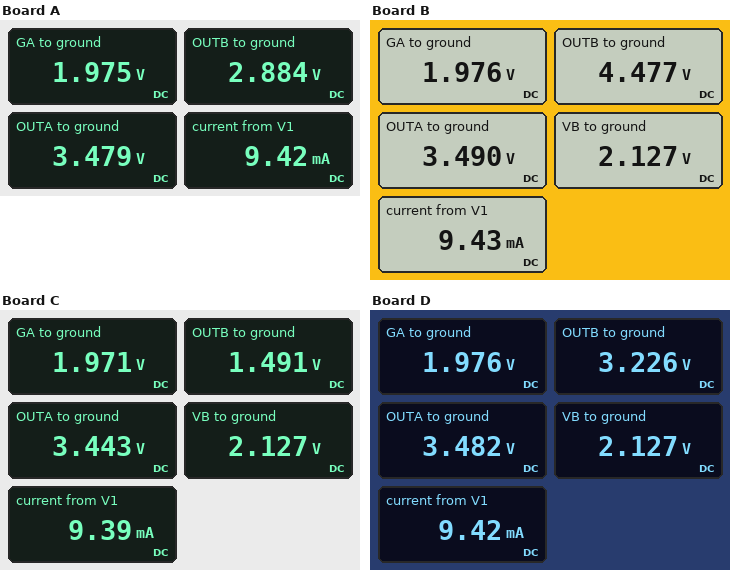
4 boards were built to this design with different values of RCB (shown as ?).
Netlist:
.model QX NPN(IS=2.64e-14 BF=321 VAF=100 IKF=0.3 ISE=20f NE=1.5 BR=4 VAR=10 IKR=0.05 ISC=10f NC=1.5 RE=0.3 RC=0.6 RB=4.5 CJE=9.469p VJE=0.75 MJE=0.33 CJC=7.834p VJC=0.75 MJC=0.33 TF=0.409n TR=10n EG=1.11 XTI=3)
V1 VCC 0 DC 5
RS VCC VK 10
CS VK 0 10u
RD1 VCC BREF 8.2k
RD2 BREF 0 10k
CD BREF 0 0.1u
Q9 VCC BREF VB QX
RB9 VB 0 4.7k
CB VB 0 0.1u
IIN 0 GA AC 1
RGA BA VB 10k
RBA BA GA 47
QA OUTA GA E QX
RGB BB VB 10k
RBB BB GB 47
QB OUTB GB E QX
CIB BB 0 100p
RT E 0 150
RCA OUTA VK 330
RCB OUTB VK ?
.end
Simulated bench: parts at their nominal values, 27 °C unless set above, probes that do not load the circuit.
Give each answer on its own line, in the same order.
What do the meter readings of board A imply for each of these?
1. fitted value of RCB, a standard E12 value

470 Ω
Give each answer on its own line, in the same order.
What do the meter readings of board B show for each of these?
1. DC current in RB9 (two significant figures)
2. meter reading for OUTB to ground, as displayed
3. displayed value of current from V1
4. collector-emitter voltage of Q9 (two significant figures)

450 µA
4.477 V
9.43 mA
2.9 V
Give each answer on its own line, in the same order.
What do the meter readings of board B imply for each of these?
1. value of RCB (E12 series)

100 Ω
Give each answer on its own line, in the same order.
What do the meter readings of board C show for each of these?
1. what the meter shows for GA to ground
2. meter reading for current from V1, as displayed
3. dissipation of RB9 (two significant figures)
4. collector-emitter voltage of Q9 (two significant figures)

1.971 V
9.39 mA
960 µW
2.9 V
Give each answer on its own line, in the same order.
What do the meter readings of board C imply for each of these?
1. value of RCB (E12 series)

820 Ω
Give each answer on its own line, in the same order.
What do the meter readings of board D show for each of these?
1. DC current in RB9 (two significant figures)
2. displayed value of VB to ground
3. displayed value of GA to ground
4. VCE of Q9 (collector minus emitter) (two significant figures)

450 µA
2.127 V
1.976 V
2.9 V
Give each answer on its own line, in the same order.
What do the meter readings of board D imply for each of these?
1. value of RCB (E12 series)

390 Ω
